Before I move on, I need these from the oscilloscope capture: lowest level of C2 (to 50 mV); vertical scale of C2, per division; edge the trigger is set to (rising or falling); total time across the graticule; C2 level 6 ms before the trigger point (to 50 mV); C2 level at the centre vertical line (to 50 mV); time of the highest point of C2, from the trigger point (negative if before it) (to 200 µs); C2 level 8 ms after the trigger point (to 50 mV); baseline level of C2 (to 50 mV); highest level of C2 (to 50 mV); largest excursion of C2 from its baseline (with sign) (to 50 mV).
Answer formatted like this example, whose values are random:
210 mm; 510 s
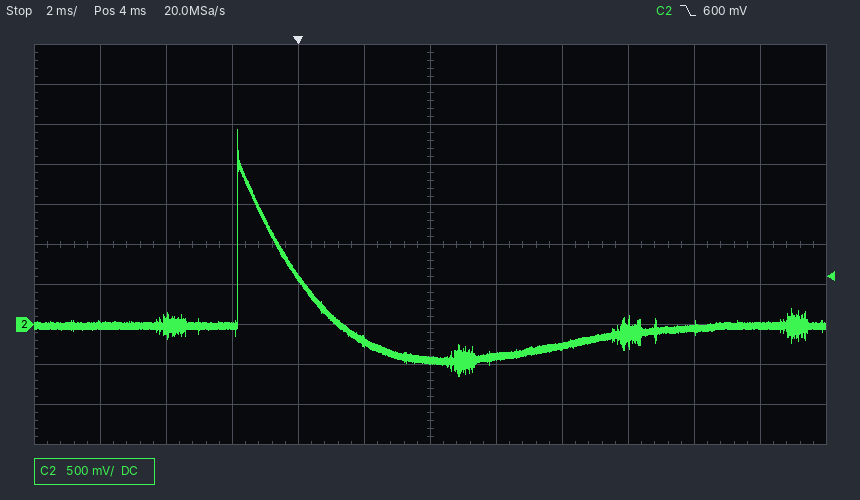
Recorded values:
-650 mV; 500 mV; falling; 24 ms; 0 mV; -450 mV; -1.8 ms; -250 mV; 0 mV; 2.45 V; +2.45 V
